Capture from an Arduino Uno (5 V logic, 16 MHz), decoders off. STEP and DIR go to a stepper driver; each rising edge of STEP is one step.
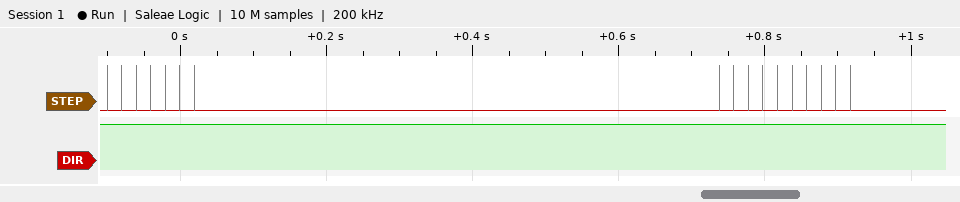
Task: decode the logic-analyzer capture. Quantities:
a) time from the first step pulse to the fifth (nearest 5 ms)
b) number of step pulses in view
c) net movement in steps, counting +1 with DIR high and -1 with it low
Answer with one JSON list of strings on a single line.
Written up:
["80 ms", "17", "+17"]
